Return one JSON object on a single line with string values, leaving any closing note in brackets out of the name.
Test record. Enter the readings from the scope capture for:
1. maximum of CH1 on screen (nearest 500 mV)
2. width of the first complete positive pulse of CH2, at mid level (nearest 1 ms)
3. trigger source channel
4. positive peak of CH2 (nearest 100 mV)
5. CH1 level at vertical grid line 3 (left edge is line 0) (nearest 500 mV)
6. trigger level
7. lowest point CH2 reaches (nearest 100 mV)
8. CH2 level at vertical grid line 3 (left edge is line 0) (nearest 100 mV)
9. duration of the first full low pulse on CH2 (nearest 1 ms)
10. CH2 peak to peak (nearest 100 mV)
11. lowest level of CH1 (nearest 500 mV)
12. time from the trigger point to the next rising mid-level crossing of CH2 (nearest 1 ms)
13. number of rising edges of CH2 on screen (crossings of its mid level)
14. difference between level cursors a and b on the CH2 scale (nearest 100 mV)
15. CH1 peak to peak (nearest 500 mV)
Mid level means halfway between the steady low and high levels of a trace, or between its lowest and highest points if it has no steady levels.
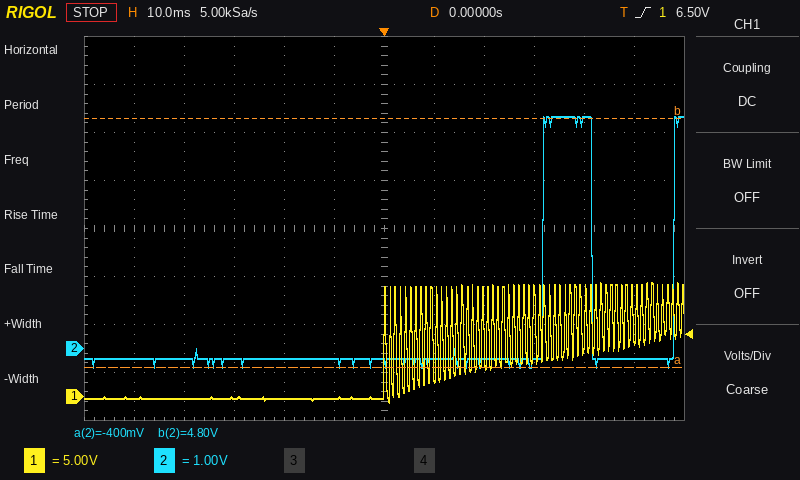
{"maximum of CH1 on screen": "12.0 V", "width of the first complete positive pulse of CH2, at mid level": "10 ms", "trigger source channel": "CH1", "positive peak of CH2": "4.8 V", "CH1 level at vertical grid line 3 (left edge is line 0)": "0.0 V", "trigger level": "6.50 V", "lowest point CH2 reaches": "-400 mV", "CH2 level at vertical grid line 3 (left edge is line 0)": "-200 mV", "duration of the first full low pulse on CH2": "16 ms", "CH2 peak to peak": "5.2 V", "lowest level of CH1": "-500 mV", "time from the trigger point to the next rising mid-level crossing of CH2": "32 ms", "number of rising edges of CH2 on screen": "2", "difference between level cursors a and b on the CH2 scale": "5.2 V", "CH1 peak to peak": "12.5 V"}
